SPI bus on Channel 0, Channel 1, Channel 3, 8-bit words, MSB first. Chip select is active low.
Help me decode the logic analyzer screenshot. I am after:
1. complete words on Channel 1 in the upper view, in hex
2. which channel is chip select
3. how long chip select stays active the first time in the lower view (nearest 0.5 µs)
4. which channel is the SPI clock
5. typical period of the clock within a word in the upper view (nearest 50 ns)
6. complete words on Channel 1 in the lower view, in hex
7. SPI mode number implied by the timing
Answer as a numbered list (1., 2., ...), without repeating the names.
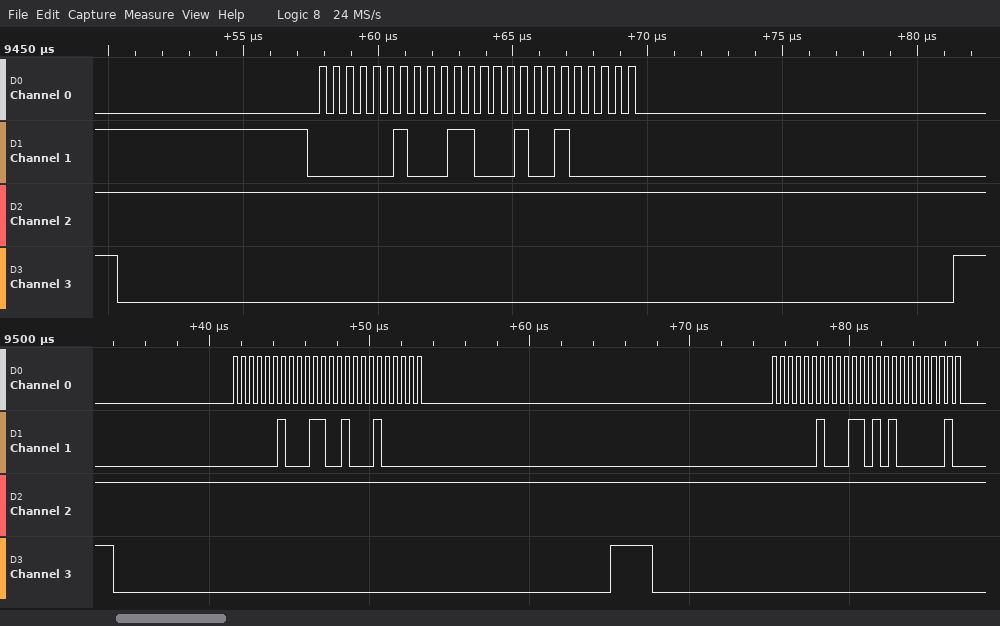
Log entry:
1. 02, 31, 20
2. Channel 3
3. 31 µs
4. Channel 0
5. 500 ns
6. 02, 32, 20, 02, 35, 02
7. 0
